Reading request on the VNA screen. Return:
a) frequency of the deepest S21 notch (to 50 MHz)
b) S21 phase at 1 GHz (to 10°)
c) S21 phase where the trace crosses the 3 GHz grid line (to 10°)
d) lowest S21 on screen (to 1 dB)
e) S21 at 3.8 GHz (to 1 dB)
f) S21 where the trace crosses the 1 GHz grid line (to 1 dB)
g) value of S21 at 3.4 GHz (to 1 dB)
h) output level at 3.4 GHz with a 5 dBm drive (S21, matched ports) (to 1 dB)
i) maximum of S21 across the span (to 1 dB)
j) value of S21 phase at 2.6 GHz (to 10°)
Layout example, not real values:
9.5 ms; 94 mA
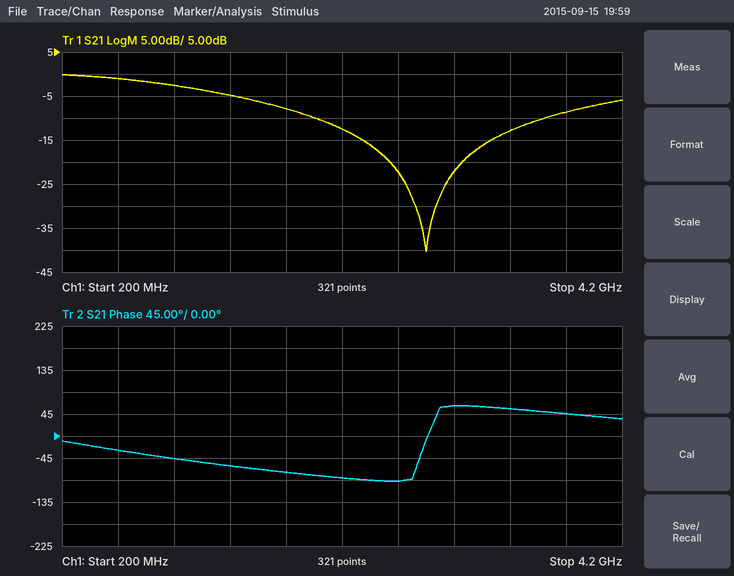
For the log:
2.80 GHz; -50°; 60°; -40 dB; -9 dB; -3 dB; -13 dB; -8 dBm; 0 dB; -90°
